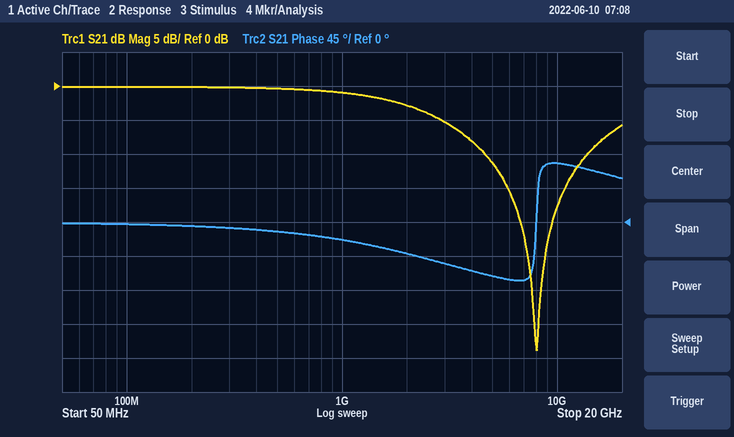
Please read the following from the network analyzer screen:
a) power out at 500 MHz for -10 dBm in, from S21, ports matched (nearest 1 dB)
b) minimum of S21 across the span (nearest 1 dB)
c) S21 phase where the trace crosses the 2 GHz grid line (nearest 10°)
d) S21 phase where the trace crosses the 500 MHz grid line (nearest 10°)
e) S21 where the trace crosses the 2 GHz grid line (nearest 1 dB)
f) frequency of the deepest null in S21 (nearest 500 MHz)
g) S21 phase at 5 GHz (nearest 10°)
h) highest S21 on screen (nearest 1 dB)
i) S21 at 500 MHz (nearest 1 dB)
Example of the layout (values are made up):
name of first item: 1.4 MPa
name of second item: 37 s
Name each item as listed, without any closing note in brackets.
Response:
power out at 500 MHz for -10 dBm in, from S21, ports matched: -10 dBm
minimum of S21 across the span: -39 dB
S21 phase where the trace crosses the 2 GHz grid line: -40°
S21 phase where the trace crosses the 500 MHz grid line: -10°
S21 where the trace crosses the 2 GHz grid line: -3 dB
frequency of the deepest null in S21: 8.0 GHz
S21 phase at 5 GHz: -70°
highest S21 on screen: 0 dB
S21 at 500 MHz: 0 dB
